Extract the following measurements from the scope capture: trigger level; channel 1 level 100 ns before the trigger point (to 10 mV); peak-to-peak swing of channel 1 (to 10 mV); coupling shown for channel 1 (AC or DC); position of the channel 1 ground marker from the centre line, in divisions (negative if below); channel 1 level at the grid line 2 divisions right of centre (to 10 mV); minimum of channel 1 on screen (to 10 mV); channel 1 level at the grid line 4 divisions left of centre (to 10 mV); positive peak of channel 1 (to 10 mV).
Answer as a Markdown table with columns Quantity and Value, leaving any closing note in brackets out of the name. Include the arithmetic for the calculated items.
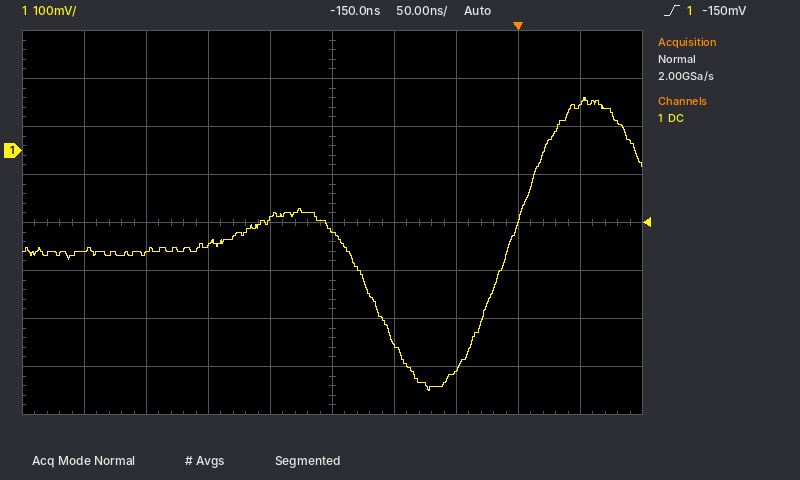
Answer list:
| Quantity | Value |
|---|---|
| trigger level | -150 mV |
| channel 1 level 100 ns before the trigger point | -400 mV |
| peak-to-peak swing of channel 1 | 110 mV − (-500 mV) = 610 mV |
| coupling shown for channel 1 | DC |
| position of the channel 1 ground marker from the centre line, in divisions | +1.5 div |
| channel 1 level at the grid line 2 divisions right of centre | -460 mV |
| minimum of channel 1 on screen | -500 mV |
| channel 1 level at the grid line 4 divisions left of centre | -210 mV |
| positive peak of channel 1 | 110 mV |
